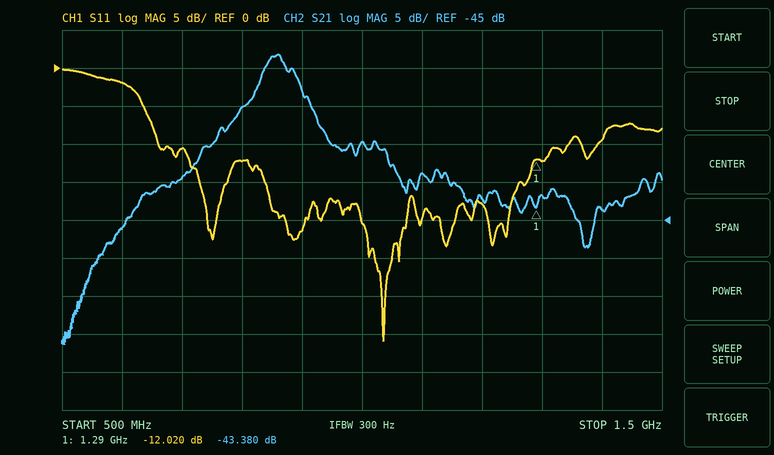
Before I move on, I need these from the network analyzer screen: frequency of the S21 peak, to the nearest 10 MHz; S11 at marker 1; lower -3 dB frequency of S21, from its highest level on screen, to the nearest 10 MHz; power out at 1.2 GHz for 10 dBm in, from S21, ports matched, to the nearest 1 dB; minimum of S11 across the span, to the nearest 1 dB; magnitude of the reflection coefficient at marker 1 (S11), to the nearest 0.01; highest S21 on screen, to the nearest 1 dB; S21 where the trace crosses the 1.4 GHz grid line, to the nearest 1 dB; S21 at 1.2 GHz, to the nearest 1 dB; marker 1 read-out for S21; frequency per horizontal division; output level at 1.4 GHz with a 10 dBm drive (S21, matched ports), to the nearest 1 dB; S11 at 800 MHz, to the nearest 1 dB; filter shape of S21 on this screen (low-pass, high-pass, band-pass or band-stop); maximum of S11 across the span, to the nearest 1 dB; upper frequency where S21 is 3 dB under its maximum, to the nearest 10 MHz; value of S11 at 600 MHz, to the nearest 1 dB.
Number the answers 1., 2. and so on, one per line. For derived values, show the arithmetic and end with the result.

1. 860 MHz
2. -12.020 dB
3. 830 MHz
4. 10 dBm + (-42 dB) = -32 dBm
5. -36 dB
6. 10^(-12.02/20) ≈ 0.25
7. -23 dB
8. -44 dB
9. -42 dB
10. -43.380 dB
11. 100 MHz
12. 10 dBm + (-44 dB) = -34 dBm
13. -12 dB
14. band-pass
15. 0 dB
16. 890 MHz
17. -2 dB
